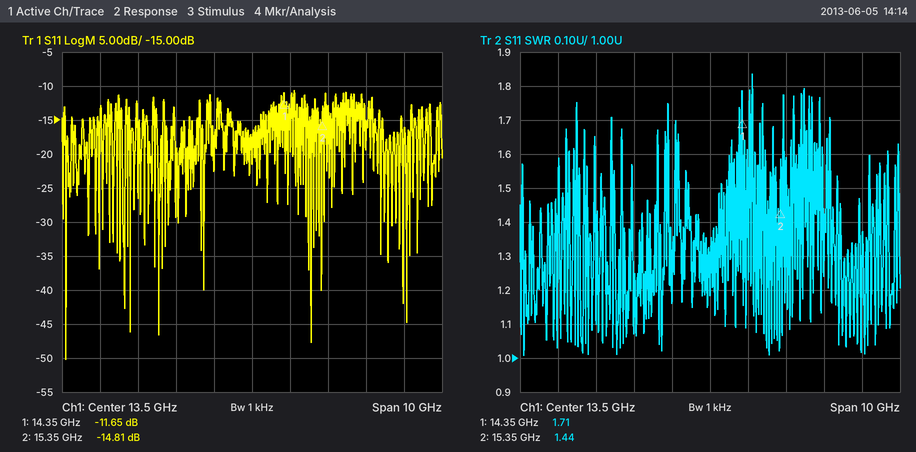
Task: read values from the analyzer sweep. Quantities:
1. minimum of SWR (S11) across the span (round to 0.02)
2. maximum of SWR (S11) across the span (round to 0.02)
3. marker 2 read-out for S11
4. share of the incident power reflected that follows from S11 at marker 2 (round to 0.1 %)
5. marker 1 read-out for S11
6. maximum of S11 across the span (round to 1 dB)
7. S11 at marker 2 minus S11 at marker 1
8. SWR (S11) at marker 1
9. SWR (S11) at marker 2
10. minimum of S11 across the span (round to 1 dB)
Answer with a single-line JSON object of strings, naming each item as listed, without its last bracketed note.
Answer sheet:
{"minimum of SWR (S11) across the span": "1.00", "maximum of SWR (S11) across the span": "1.84", "marker 2 read-out for S11": "-14.81 dB", "share of the incident power reflected that follows from S11 at marker 2": "3.3 %", "marker 1 read-out for S11": "-11.65 dB", "maximum of S11 across the span": "-11 dB", "S11 at marker 2 minus S11 at marker 1": "-3.16 dB", "SWR (S11) at marker 1": "1.71", "SWR (S11) at marker 2": "1.44", "minimum of S11 across the span": "-50 dB"}
